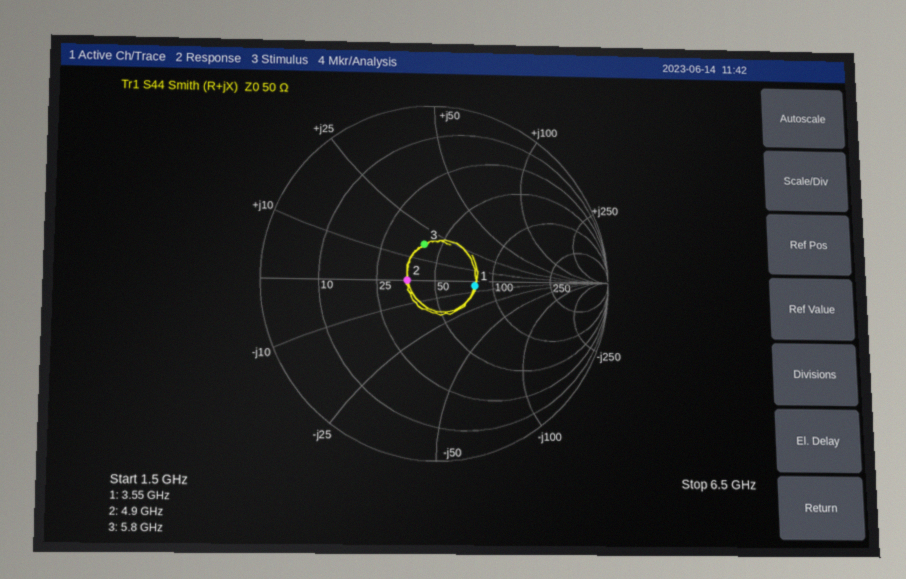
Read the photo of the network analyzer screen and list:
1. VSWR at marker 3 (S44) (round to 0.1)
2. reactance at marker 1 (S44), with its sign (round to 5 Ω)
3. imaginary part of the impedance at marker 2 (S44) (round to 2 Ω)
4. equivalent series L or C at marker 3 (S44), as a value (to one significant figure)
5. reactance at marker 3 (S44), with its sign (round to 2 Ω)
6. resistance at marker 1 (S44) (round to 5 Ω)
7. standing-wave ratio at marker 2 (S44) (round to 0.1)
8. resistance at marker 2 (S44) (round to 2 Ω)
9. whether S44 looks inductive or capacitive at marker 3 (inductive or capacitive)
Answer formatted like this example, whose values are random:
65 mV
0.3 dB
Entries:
1.5
-5 Ω
0 Ω
500 pH
+18 Ω
80 Ω
1.4
36 Ω
inductive
